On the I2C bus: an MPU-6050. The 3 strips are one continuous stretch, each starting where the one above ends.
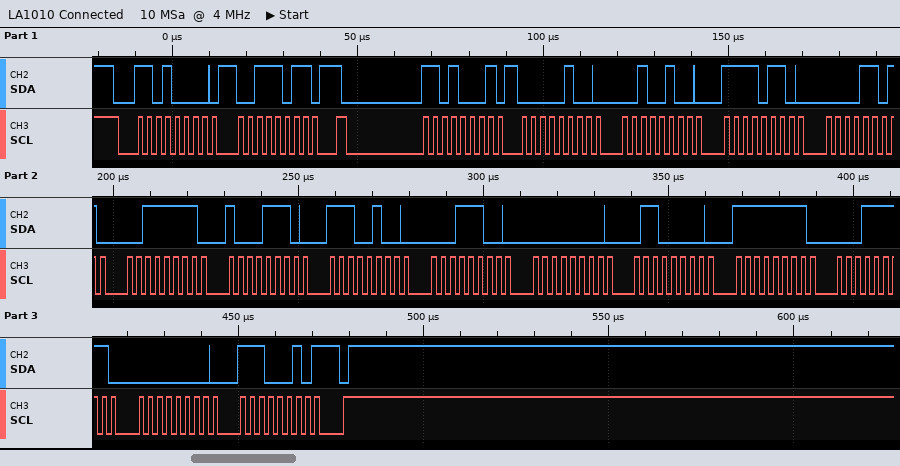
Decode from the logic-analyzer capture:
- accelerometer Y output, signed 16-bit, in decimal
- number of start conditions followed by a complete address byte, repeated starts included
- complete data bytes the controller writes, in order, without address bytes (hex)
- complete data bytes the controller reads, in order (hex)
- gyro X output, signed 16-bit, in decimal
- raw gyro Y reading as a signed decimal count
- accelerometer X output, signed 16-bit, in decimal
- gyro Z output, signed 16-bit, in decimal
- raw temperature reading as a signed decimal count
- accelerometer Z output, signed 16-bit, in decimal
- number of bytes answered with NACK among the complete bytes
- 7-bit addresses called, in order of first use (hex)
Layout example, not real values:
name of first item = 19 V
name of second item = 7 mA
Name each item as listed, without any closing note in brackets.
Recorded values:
accelerometer Y output, signed 16-bit, in decimal = -2547
number of start conditions followed by a complete address byte, repeated starts included = 2
complete data bytes the controller writes, in order, without address bytes = 3B
complete data bytes the controller reads, in order = 04 24 F6 0D 3F 8E E4 1C 00 60 FF 1F 00 E2
gyro X output, signed 16-bit, in decimal = 96
raw gyro Y reading as a signed decimal count = -225
accelerometer X output, signed 16-bit, in decimal = 1060
gyro Z output, signed 16-bit, in decimal = 226
raw temperature reading as a signed decimal count = -7140
accelerometer Z output, signed 16-bit, in decimal = 16270
number of bytes answered with NACK among the complete bytes = 1
7-bit addresses called, in order of first use = 0x68
